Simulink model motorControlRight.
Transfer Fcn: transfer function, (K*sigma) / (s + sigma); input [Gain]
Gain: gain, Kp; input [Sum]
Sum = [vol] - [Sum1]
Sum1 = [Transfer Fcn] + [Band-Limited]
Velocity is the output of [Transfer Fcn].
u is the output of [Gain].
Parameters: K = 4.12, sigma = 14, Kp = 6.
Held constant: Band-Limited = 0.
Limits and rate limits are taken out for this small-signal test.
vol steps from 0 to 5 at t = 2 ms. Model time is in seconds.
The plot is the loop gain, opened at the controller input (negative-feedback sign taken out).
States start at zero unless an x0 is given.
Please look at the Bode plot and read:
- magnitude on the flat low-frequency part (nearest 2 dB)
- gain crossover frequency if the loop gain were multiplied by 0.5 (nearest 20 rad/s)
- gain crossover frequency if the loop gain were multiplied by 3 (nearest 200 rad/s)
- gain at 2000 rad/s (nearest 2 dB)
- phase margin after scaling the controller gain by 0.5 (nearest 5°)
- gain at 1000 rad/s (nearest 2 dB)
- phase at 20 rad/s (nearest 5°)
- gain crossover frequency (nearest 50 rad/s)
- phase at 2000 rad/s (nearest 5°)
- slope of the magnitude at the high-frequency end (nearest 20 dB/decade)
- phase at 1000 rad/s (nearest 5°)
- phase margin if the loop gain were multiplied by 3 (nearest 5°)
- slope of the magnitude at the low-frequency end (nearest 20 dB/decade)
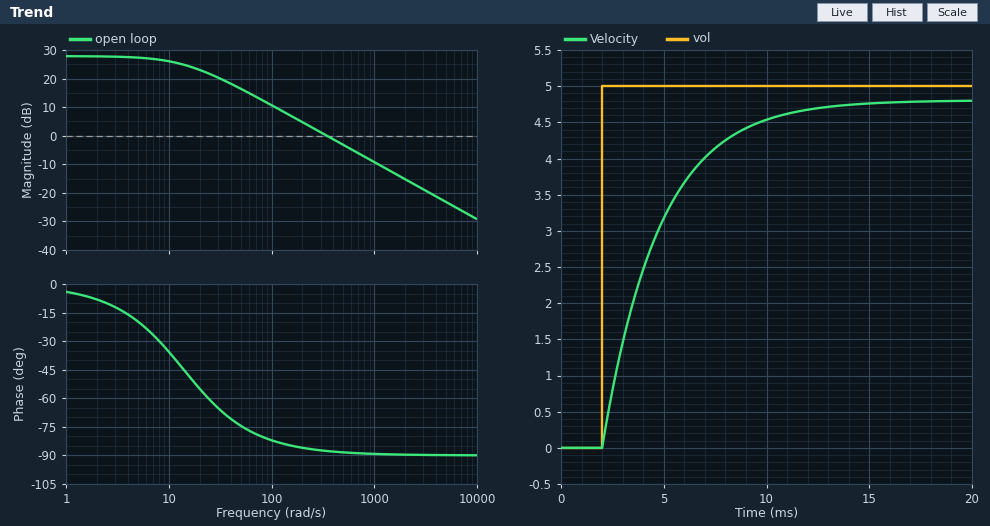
28 dB
180 rad/s
1000 rad/s
-16 dB
95°
-10 dB
-55°
350 rad/s
-90°
-20 dB/decade
-90°
90°
0 dB/decade
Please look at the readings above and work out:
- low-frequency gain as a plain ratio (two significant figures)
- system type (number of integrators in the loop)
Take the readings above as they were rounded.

25
0
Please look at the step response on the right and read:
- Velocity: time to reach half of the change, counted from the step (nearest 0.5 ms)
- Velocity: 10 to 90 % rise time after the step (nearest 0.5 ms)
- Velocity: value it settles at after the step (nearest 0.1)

2.0 ms
6.0 ms
4.8
